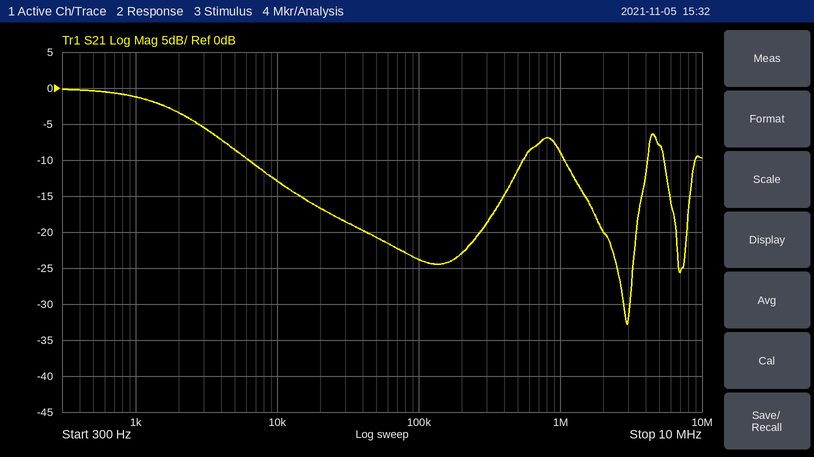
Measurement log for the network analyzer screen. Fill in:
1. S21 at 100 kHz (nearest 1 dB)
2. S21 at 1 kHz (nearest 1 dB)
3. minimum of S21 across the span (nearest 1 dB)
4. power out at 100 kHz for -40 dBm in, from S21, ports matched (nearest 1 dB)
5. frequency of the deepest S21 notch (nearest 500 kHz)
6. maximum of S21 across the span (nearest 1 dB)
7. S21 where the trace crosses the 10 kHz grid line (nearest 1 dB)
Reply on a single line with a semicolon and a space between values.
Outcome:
-24 dB; -1 dB; -33 dB; -64 dBm; 3.0 MHz; 0 dB; -13 dB
